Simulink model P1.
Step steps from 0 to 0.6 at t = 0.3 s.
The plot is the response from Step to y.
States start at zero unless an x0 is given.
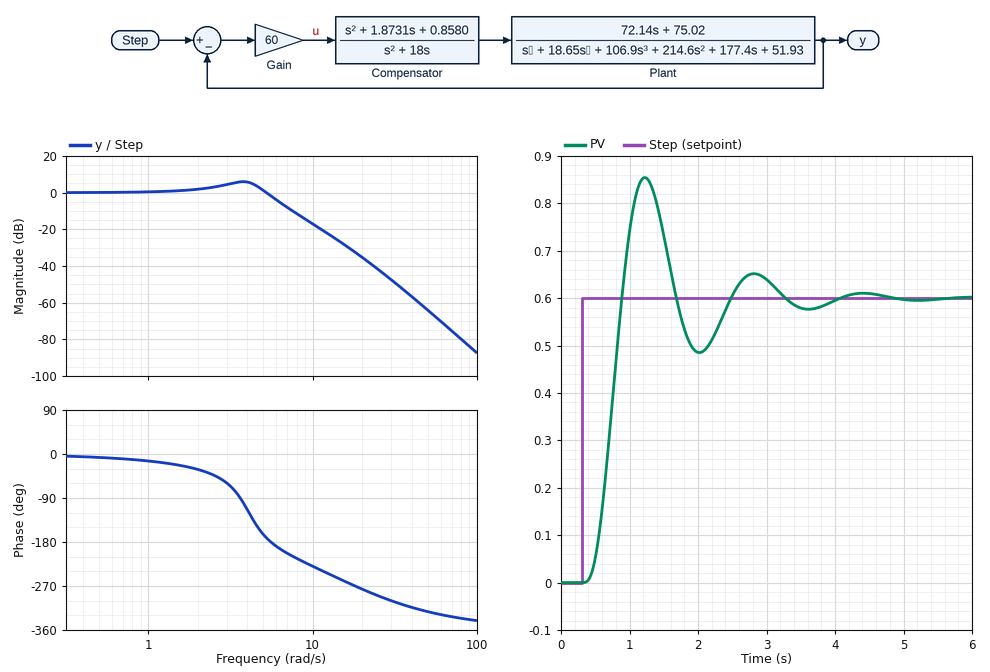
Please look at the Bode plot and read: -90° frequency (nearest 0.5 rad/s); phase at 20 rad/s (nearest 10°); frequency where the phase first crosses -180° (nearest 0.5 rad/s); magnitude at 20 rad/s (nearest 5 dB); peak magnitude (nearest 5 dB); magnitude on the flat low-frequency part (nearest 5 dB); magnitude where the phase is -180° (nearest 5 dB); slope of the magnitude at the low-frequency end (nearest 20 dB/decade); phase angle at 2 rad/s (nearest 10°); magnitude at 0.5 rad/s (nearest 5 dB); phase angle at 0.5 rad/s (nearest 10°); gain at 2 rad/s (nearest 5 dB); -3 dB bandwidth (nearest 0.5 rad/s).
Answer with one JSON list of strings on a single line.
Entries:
["3.5 rad/s", "-280°", "5.5 rad/s", "-35 dB", "5 dB", "0 dB", "0 dB", "0 dB/decade", "-30°", "0 dB", "-10°", "0 dB", "6.0 rad/s"]
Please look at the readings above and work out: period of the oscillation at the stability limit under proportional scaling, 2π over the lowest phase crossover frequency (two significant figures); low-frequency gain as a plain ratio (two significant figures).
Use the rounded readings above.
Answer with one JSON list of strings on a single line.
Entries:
["1.1 s", "1.0"]
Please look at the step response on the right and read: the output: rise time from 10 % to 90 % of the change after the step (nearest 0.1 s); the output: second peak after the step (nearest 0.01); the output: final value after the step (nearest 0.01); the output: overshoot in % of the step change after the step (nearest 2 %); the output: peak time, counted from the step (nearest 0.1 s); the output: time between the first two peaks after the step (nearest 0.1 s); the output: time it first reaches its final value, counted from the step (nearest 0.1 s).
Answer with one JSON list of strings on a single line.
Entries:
["0.3 s", "0.65", "0.60", "42 %", "0.9 s", "1.6 s", "0.6 s"]
